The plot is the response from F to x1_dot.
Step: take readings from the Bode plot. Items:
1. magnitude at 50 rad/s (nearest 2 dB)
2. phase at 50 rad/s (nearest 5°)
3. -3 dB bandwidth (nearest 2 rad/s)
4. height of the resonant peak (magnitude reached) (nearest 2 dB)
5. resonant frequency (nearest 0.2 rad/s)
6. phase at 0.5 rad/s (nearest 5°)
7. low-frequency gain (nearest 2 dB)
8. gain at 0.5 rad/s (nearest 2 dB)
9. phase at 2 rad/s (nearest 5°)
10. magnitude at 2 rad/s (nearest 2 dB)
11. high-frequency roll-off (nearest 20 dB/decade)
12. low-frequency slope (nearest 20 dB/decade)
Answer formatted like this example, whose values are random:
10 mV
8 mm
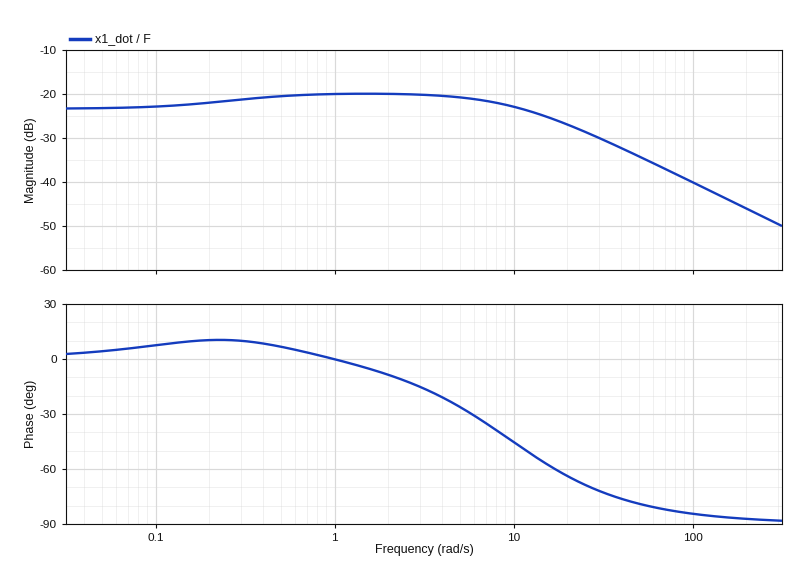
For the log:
-34 dB
-80°
18 rad/s
-20 dB
1.4 rad/s
5°
-24 dB
-20 dB
-10°
-20 dB
-20 dB/decade
0 dB/decade
